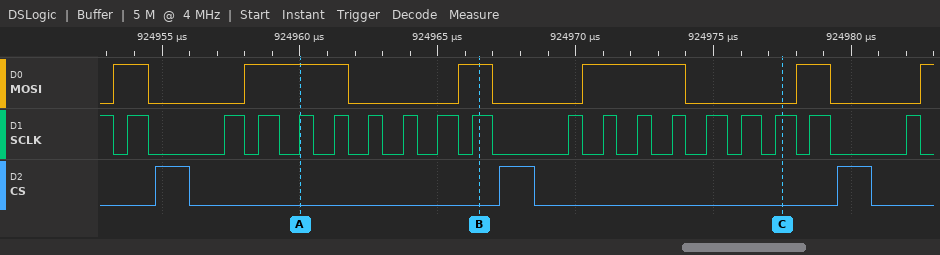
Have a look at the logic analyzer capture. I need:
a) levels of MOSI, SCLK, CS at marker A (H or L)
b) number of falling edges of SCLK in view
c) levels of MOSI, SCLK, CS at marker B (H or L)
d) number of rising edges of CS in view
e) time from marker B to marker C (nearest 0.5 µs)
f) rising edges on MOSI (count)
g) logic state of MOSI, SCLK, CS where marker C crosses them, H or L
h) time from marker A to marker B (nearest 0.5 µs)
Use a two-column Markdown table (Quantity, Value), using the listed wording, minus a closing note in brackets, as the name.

| Quantity | Value |
|---|---|
| levels of MOSI, SCLK, CS at marker A | MOSI=H, SCLK=H, CS=L |
| number of falling edges of SCLK in view | 19 |
| levels of MOSI, SCLK, CS at marker B | MOSI=H, SCLK=H, CS=L |
| number of rising edges of CS in view | 3 |
| time from marker B to marker C | 11 µs |
| rising edges on MOSI | 6 |
| logic state of MOSI, SCLK, CS where marker C crosses them, H or L | MOSI=L, SCLK=H, CS=L |
| time from marker A to marker B | 6.5 µs |
